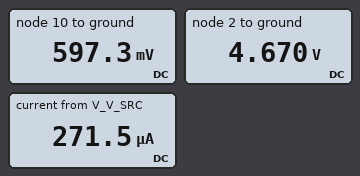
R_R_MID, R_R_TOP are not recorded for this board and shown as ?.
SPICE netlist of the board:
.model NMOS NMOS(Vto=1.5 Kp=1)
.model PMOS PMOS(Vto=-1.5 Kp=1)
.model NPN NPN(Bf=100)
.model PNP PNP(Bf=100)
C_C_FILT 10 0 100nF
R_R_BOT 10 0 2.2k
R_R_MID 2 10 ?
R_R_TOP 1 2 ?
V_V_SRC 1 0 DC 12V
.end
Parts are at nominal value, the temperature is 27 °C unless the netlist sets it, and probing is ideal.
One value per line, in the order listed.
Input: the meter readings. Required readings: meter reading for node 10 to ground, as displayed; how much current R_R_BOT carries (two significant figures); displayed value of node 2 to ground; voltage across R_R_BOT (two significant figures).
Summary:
597.3 mV
270 µA
4.670 V
600 mV
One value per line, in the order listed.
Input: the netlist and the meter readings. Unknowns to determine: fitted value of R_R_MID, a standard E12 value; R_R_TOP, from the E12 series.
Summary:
15 kΩ
27 kΩ
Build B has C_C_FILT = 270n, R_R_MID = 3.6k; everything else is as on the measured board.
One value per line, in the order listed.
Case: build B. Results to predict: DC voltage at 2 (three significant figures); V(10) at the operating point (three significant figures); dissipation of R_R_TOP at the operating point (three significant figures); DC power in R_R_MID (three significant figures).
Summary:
2.12 V
805 mV
3.61 mW
482 µW
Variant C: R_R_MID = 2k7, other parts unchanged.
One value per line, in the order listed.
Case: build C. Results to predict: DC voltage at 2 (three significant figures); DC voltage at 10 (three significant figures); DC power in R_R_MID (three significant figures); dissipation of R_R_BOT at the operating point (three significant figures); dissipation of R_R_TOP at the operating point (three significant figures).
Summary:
1.84 V
828 mV
382 µW
311 µW
3.82 mW
